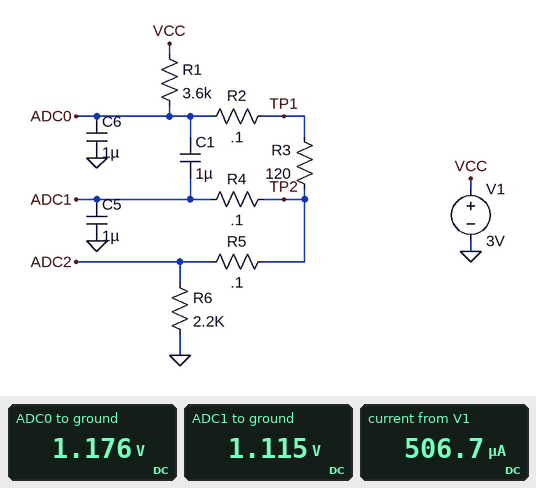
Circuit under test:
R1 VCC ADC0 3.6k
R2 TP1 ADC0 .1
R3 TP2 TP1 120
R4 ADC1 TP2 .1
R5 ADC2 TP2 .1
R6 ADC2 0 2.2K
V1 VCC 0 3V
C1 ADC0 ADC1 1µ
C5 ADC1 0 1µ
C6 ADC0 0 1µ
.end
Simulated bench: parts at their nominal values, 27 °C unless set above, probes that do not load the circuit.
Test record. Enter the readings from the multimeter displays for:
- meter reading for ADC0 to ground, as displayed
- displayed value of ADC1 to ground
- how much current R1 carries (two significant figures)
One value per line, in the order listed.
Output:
1.176 V
1.115 V
510 µA
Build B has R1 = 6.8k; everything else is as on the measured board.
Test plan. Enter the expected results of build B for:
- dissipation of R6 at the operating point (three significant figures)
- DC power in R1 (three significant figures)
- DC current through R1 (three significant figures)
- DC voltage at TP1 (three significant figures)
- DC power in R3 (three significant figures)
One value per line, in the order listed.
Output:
238 µW
736 µW
329 µA
763 mV
13.0 µW
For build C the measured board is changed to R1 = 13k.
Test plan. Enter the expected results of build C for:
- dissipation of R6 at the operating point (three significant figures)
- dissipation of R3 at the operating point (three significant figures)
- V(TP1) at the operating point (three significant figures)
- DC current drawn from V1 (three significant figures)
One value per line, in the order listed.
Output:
84.4 µW
4.60 µW
454 mV
196 µA
